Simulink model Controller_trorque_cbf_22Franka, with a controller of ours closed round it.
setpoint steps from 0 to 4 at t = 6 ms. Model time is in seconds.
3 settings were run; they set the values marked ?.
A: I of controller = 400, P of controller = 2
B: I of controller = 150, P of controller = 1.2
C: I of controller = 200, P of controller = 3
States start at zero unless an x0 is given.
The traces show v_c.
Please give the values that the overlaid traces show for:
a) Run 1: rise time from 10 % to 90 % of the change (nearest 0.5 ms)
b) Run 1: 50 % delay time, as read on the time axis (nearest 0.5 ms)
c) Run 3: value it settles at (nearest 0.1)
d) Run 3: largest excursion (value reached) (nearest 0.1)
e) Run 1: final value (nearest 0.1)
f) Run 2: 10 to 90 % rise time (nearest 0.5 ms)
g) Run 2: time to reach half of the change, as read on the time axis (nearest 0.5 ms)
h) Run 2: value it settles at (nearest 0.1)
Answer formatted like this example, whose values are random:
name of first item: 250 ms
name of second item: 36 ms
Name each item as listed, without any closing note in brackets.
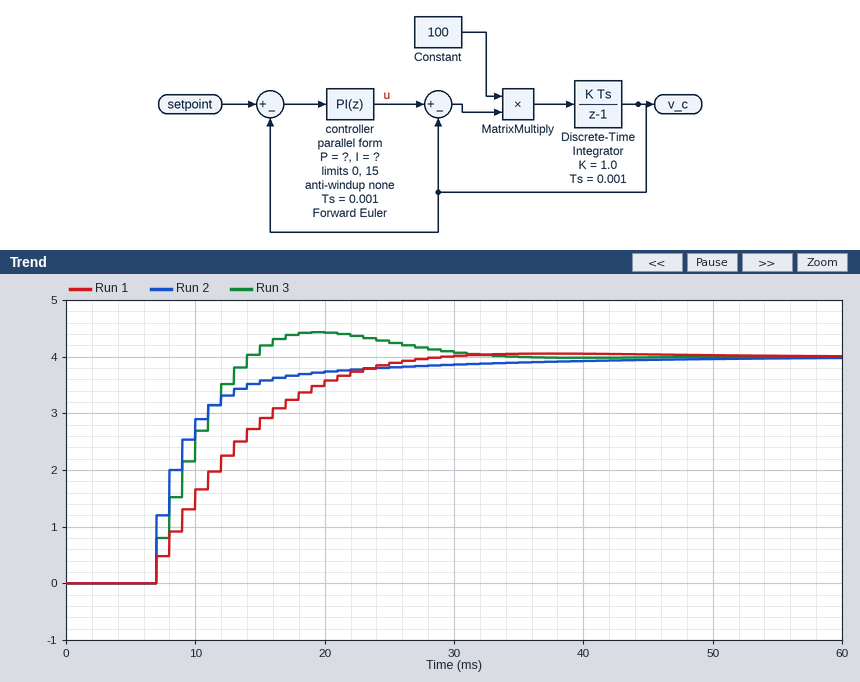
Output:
Run 1: rise time from 10 % to 90 % of the change: 14.0 ms
Run 1: 50 % delay time, as read on the time axis: 12.0 ms
Run 3: value it settles at: 4.0
Run 3: largest excursion (value reached): 4.4
Run 1: final value: 4.0
Run 2: 10 to 90 % rise time: 9.0 ms
Run 2: time to reach half of the change, as read on the time axis: 8.0 ms
Run 2: value it settles at: 4.0
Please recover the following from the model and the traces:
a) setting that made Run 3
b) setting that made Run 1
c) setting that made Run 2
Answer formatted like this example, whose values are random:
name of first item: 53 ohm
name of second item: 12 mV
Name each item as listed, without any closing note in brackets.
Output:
setting that made Run 3: A
setting that made Run 1: B
setting that made Run 2: C
